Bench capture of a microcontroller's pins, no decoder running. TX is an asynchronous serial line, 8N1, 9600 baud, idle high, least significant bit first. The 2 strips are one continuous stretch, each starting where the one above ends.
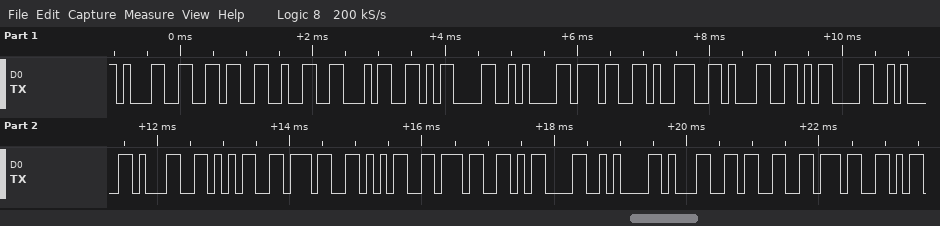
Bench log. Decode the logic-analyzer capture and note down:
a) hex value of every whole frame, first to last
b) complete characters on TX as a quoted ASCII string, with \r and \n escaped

0x31 0x36 0x32 0x34 0x0D 0x0A 0x37 0x39 0x31 0x0D 0x0A 0x31 0x35 0x37 0x35 0x37 0x0D 0x0A 0x31 0x33 0x37
"1624\r\n791\r\n15757\r\n137"
